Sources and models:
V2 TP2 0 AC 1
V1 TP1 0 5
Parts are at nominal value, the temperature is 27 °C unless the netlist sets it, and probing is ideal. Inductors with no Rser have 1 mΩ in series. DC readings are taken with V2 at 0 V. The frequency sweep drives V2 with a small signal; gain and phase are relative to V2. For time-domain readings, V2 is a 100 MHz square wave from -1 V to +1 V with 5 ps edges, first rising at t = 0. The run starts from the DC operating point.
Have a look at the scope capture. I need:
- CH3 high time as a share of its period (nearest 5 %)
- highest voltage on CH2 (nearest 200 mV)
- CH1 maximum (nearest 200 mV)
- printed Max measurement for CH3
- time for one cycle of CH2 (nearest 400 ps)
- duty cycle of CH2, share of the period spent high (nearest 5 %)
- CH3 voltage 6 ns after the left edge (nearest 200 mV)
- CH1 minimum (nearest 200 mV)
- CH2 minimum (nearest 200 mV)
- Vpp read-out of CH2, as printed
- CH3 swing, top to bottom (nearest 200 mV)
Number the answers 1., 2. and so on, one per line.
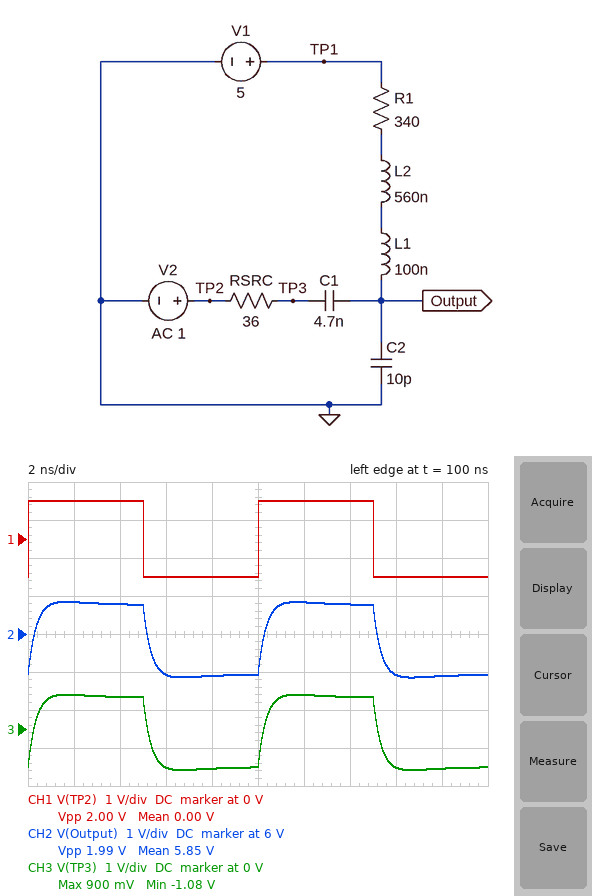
1. 50 %
2. 6.8 V
3. 1.0 V
4. 900 mV
5. 10.0 ns
6. 50 %
7. -1.0 V
8. -1.0 V
9. 4.8 V
10. 1.99 V
11. 2.0 V
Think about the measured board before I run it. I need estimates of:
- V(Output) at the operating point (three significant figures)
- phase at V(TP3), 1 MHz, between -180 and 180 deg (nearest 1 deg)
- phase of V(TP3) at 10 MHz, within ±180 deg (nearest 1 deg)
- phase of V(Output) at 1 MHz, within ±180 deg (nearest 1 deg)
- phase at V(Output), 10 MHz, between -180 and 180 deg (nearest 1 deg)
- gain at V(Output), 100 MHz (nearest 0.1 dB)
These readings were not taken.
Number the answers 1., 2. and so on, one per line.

1. 5.00 V
2. -1 deg
3. -1 deg
4. 5 deg
5. 0 deg
6. -0.5 dB
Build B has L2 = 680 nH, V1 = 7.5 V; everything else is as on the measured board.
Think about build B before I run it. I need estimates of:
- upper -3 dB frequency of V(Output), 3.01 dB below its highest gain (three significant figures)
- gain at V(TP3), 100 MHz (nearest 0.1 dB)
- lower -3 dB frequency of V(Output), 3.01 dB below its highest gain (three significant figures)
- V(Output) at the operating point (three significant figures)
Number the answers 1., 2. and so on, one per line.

1. 491 MHz
2. -0.4 dB
3. 100 kHz
4. 7.50 V
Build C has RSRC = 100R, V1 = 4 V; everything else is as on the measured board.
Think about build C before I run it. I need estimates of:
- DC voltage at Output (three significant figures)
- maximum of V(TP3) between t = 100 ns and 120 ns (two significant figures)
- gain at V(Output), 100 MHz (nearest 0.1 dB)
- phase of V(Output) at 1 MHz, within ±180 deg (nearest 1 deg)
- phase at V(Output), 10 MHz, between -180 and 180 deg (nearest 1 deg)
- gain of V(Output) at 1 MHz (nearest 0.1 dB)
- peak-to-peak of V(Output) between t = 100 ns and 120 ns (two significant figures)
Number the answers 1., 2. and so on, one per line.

1. 4.00 V
2. 680 mV
3. -1.7 dB
4. 4 deg
5. -1 deg
6. -2.3 dB
7. 1.8 V
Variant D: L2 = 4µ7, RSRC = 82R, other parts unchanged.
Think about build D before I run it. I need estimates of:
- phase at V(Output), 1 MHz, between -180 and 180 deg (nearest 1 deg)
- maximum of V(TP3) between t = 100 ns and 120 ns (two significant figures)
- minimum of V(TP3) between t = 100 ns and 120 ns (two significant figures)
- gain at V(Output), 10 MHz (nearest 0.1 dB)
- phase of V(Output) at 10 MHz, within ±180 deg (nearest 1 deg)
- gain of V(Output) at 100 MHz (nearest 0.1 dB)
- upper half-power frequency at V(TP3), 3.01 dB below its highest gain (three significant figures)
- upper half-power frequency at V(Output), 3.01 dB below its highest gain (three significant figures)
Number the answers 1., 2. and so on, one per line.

1. 5 deg
2. 800 mV
3. -1.2 V
4. -1.1 dB
5. 4 deg
6. -1.0 dB
7. 197 MHz
8. 207 MHz
